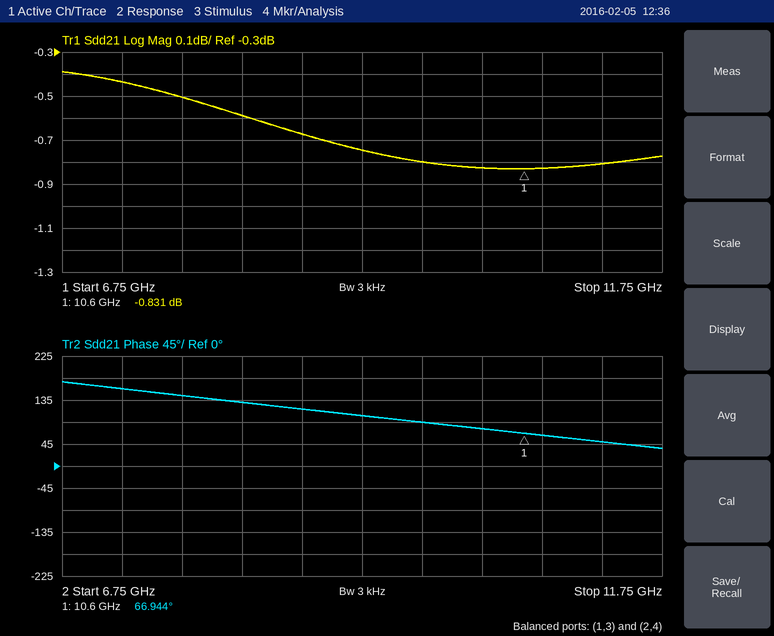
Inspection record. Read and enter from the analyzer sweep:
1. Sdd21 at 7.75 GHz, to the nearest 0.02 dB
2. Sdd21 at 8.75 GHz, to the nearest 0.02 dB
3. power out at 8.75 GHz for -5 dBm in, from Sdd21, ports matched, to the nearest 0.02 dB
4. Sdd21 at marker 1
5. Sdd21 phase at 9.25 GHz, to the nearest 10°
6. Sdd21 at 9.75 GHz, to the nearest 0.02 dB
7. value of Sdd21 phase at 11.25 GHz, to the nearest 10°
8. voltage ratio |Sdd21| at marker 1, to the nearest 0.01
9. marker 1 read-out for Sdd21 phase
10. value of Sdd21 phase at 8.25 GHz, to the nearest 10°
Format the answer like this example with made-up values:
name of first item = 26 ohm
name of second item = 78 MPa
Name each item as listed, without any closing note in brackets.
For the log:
Sdd21 at 7.75 GHz, to the nearest 0.02 dB = -0.50 dB
Sdd21 at 8.75 GHz, to the nearest 0.02 dB = -0.68 dB
power out at 8.75 GHz for -5 dBm in, from Sdd21, ports matched, to the nearest 0.02 dB = -5.68 dBm
Sdd21 at marker 1 = -0.831 dB
Sdd21 phase at 9.25 GHz, to the nearest 10° = 100°
Sdd21 at 9.75 GHz, to the nearest 0.02 dB = -0.80 dB
value of Sdd21 phase at 11.25 GHz, to the nearest 10° = 50°
voltage ratio |Sdd21| at marker 1, to the nearest 0.01 = 0.91
marker 1 read-out for Sdd21 phase = 66.944°
value of Sdd21 phase at 8.25 GHz, to the nearest 10° = 130°
